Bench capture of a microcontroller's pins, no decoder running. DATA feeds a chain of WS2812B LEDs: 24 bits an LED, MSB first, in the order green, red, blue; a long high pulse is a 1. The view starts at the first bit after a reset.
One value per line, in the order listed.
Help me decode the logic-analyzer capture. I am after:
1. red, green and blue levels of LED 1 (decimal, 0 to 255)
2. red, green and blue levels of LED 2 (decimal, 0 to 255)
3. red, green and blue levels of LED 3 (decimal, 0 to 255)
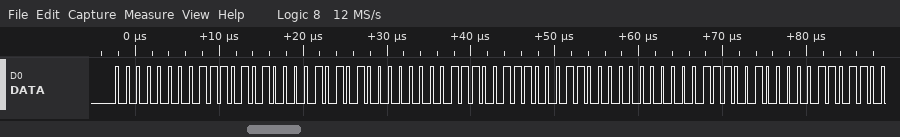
234, 0, 21
231, 0, 24
228, 0, 27
